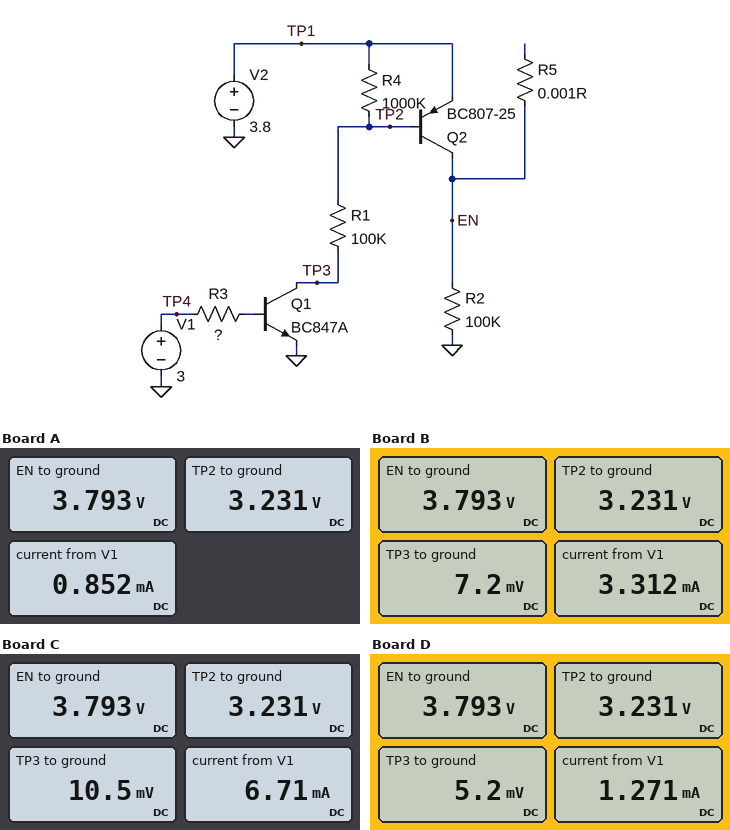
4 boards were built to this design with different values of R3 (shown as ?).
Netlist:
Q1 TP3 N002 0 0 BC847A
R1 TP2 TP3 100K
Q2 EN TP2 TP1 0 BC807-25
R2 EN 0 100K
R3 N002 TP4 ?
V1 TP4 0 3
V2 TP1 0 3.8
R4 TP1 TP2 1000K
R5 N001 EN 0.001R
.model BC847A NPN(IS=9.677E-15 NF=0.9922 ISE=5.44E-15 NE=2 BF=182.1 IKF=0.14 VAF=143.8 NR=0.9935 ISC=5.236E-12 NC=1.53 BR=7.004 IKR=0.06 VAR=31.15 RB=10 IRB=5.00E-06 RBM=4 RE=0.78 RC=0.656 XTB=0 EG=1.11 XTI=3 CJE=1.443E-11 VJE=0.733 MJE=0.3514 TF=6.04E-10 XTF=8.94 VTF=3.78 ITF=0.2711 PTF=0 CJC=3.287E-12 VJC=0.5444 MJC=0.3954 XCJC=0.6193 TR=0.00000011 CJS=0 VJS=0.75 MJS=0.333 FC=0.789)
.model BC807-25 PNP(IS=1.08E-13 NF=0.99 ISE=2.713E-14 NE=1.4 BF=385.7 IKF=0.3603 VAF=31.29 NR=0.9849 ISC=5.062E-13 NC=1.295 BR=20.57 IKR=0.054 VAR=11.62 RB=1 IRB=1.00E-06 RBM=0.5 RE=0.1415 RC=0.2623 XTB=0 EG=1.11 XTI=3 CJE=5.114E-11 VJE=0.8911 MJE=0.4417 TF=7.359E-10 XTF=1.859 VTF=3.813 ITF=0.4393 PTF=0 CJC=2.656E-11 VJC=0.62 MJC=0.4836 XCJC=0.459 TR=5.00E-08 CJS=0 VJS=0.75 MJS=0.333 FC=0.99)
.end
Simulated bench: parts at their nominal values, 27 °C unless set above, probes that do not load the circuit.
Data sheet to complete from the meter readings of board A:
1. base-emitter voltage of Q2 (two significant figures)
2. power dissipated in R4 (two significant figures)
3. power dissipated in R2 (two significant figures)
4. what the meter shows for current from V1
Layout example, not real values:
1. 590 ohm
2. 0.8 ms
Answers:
1. -570 mV
2. 320 nW
3. 140 µW
4. 0.852 mA
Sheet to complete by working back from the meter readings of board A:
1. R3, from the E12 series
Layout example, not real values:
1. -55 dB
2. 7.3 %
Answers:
1. 2.7 kΩ
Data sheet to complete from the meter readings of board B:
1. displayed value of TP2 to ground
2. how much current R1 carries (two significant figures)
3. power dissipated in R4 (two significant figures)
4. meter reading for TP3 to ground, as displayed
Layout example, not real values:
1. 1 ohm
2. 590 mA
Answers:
1. 3.231 V
2. 32 µA
3. 320 nW
4. 7.2 mV
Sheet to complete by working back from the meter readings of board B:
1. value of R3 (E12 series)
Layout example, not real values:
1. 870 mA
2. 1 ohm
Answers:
1. 680 Ω
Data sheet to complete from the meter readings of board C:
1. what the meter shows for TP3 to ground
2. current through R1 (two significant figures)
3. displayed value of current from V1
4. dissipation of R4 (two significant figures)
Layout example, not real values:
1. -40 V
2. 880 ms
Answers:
1. 10.5 mV
2. 32 µA
3. 6.71 mA
4. 320 nW
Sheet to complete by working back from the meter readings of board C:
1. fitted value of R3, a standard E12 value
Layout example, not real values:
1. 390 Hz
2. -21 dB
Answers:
1. 330 Ω
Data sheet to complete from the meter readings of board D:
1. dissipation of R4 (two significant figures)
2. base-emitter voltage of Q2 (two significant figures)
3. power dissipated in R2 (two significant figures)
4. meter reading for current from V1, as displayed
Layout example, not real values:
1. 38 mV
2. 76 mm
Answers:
1. 320 nW
2. -570 mV
3. 140 µW
4. 1.271 mA
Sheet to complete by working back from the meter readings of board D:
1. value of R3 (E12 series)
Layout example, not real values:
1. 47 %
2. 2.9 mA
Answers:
1. 1.8 kΩ
